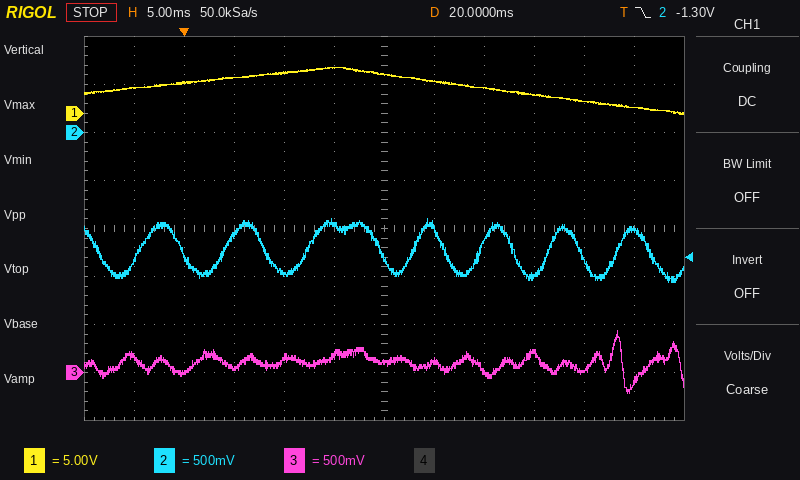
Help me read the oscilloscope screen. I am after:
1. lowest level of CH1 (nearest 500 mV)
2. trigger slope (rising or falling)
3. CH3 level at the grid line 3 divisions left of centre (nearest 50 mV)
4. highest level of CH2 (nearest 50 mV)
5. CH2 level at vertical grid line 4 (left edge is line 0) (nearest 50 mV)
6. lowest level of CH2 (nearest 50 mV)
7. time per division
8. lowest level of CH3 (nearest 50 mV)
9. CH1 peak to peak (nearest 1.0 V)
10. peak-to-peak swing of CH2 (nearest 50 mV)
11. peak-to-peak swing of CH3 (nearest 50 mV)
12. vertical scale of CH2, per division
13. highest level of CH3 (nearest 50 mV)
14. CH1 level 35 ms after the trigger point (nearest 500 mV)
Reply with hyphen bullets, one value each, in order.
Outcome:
- 0.0 V
- falling
- 50 mV
- -900 mV
- -1.45 V
- -1.55 V
- 5 ms
- -200 mV
- 5.0 V
- 650 mV
- 650 mV
- 500 mV
- 450 mV
- 2.0 V
